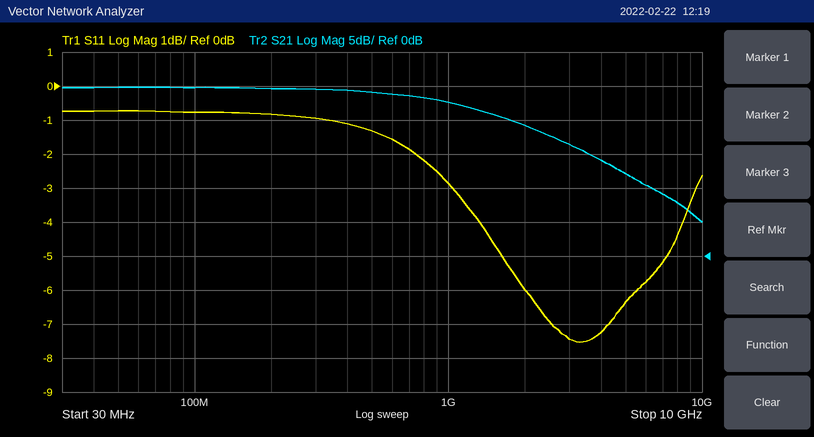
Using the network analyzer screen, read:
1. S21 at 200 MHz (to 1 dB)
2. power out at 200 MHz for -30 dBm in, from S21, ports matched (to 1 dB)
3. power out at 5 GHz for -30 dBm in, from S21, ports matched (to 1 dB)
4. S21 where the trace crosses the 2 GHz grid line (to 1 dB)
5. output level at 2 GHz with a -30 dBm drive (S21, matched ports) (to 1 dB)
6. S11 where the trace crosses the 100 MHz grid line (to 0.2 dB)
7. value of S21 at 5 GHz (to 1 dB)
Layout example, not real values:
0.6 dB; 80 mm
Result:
25 dB; -5 dBm; -18 dBm; 19 dB; -11 dBm; -0.8 dB; 12 dB
